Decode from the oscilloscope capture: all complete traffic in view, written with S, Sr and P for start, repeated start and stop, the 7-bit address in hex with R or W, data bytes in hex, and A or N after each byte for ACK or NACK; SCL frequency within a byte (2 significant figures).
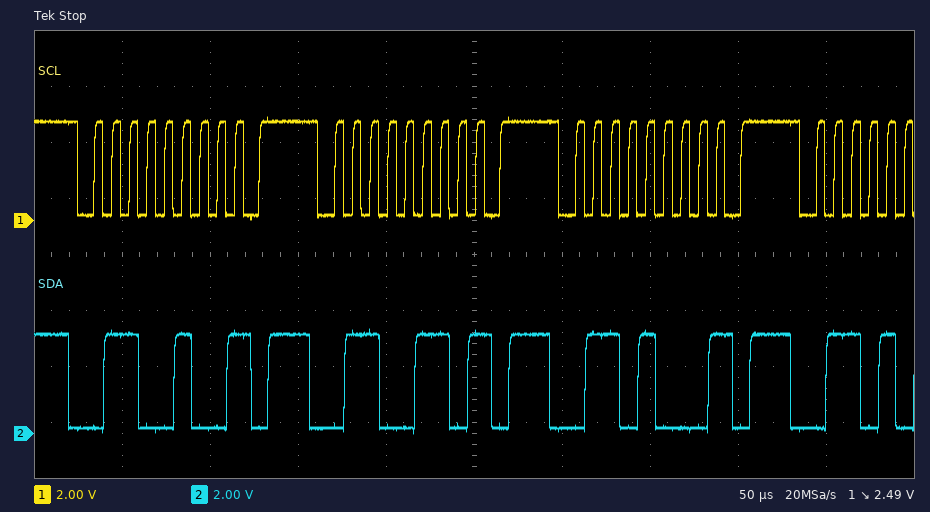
S 32W N P S 33W N P S 34W N P
100 kHz
